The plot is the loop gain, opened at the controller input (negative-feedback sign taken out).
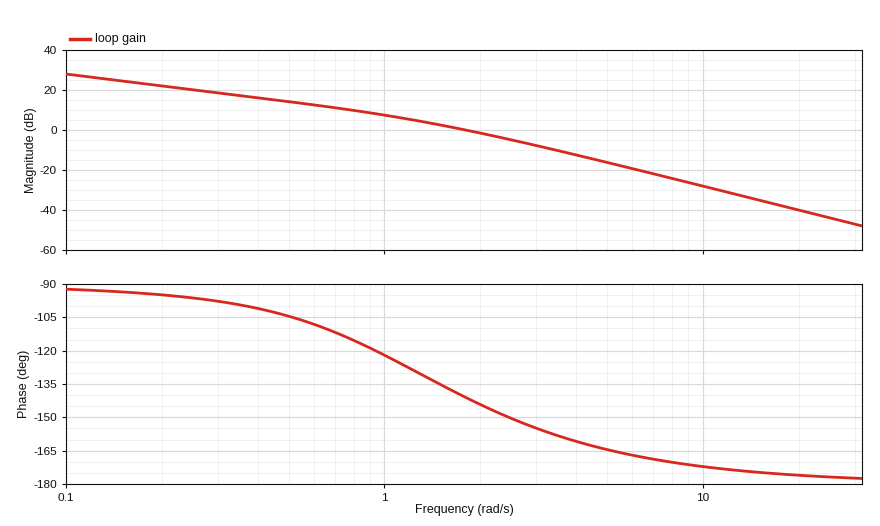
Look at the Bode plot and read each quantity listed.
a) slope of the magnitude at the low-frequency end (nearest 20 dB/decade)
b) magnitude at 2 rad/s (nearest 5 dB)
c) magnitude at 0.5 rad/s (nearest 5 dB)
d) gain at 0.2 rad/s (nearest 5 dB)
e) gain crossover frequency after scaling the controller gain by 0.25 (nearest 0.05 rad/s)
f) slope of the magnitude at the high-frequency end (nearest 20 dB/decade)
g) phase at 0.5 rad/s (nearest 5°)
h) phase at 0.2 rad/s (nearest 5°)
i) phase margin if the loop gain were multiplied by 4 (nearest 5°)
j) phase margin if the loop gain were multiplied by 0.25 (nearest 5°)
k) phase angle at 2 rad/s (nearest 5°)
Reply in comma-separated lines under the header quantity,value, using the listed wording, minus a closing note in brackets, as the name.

quantity,value
slope of the magnitude at the low-frequency end,-20 dB/decade
magnitude at 2 rad/s,0 dB
magnitude at 0.5 rad/s,15 dB
gain at 0.2 rad/s,20 dB
gain crossover frequency after scaling the controller gain by 0.25,0.65 rad/s
slope of the magnitude at the high-frequency end,-40 dB/decade
phase at 0.5 rad/s,-105°
phase at 0.2 rad/s,-95°
phase margin if the loop gain were multiplied by 4,20°
phase margin if the loop gain were multiplied by 0.25,70°
phase angle at 2 rad/s,-145°
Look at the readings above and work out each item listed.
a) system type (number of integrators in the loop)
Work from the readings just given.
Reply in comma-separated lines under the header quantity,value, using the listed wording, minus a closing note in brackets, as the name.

quantity,value
system type,1
